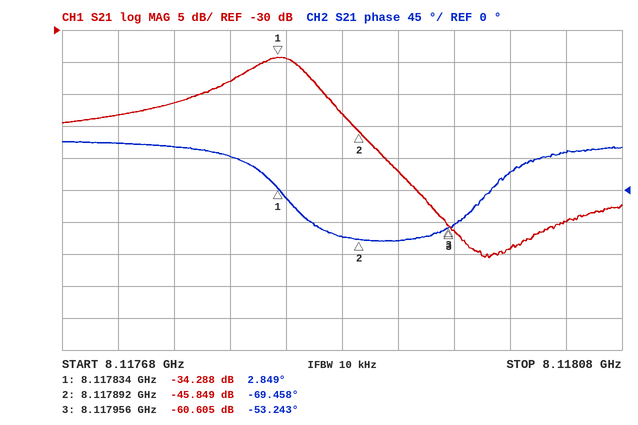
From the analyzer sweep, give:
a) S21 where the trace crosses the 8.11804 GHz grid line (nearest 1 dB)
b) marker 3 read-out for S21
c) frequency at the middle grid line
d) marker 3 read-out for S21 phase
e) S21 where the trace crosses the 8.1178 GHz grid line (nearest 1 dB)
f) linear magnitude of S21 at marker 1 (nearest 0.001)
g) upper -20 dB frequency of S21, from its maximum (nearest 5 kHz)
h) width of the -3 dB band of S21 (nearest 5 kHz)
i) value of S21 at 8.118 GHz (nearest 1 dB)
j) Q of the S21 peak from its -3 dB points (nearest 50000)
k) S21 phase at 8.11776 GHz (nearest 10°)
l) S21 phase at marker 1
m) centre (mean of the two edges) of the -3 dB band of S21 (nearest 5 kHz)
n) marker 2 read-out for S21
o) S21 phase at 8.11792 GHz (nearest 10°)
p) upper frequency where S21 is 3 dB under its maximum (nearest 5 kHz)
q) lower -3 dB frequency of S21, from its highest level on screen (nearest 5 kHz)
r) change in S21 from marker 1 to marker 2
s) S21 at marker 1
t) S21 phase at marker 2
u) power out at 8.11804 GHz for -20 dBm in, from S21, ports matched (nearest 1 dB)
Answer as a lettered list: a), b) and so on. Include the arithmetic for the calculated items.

a) -60 dB
b) -60.605 dB
c) 8.11788 GHz
d) -53.243°
e) -38 dB
f) 10^(-34.288/20) ≈ 0.019
g) 8.117930 GHz
h) 8.117855 GHz − 8.117805 GHz = 50 kHz
i) -64 dB
j) 8.11783 GHz / 50 kHz ≈ 162357, so 150000 to the nearest 50000
k) 60°
l) 2.849°
m) 8.117830 GHz
n) -45.849 dB
o) -70°
p) 8.117855 GHz
q) 8.117805 GHz
r) -45.849 − (-34.288) = -11.561 dB
s) -34.288 dB
t) -69.458°
u) -20 dBm + (-60 dB) = -80 dBm
